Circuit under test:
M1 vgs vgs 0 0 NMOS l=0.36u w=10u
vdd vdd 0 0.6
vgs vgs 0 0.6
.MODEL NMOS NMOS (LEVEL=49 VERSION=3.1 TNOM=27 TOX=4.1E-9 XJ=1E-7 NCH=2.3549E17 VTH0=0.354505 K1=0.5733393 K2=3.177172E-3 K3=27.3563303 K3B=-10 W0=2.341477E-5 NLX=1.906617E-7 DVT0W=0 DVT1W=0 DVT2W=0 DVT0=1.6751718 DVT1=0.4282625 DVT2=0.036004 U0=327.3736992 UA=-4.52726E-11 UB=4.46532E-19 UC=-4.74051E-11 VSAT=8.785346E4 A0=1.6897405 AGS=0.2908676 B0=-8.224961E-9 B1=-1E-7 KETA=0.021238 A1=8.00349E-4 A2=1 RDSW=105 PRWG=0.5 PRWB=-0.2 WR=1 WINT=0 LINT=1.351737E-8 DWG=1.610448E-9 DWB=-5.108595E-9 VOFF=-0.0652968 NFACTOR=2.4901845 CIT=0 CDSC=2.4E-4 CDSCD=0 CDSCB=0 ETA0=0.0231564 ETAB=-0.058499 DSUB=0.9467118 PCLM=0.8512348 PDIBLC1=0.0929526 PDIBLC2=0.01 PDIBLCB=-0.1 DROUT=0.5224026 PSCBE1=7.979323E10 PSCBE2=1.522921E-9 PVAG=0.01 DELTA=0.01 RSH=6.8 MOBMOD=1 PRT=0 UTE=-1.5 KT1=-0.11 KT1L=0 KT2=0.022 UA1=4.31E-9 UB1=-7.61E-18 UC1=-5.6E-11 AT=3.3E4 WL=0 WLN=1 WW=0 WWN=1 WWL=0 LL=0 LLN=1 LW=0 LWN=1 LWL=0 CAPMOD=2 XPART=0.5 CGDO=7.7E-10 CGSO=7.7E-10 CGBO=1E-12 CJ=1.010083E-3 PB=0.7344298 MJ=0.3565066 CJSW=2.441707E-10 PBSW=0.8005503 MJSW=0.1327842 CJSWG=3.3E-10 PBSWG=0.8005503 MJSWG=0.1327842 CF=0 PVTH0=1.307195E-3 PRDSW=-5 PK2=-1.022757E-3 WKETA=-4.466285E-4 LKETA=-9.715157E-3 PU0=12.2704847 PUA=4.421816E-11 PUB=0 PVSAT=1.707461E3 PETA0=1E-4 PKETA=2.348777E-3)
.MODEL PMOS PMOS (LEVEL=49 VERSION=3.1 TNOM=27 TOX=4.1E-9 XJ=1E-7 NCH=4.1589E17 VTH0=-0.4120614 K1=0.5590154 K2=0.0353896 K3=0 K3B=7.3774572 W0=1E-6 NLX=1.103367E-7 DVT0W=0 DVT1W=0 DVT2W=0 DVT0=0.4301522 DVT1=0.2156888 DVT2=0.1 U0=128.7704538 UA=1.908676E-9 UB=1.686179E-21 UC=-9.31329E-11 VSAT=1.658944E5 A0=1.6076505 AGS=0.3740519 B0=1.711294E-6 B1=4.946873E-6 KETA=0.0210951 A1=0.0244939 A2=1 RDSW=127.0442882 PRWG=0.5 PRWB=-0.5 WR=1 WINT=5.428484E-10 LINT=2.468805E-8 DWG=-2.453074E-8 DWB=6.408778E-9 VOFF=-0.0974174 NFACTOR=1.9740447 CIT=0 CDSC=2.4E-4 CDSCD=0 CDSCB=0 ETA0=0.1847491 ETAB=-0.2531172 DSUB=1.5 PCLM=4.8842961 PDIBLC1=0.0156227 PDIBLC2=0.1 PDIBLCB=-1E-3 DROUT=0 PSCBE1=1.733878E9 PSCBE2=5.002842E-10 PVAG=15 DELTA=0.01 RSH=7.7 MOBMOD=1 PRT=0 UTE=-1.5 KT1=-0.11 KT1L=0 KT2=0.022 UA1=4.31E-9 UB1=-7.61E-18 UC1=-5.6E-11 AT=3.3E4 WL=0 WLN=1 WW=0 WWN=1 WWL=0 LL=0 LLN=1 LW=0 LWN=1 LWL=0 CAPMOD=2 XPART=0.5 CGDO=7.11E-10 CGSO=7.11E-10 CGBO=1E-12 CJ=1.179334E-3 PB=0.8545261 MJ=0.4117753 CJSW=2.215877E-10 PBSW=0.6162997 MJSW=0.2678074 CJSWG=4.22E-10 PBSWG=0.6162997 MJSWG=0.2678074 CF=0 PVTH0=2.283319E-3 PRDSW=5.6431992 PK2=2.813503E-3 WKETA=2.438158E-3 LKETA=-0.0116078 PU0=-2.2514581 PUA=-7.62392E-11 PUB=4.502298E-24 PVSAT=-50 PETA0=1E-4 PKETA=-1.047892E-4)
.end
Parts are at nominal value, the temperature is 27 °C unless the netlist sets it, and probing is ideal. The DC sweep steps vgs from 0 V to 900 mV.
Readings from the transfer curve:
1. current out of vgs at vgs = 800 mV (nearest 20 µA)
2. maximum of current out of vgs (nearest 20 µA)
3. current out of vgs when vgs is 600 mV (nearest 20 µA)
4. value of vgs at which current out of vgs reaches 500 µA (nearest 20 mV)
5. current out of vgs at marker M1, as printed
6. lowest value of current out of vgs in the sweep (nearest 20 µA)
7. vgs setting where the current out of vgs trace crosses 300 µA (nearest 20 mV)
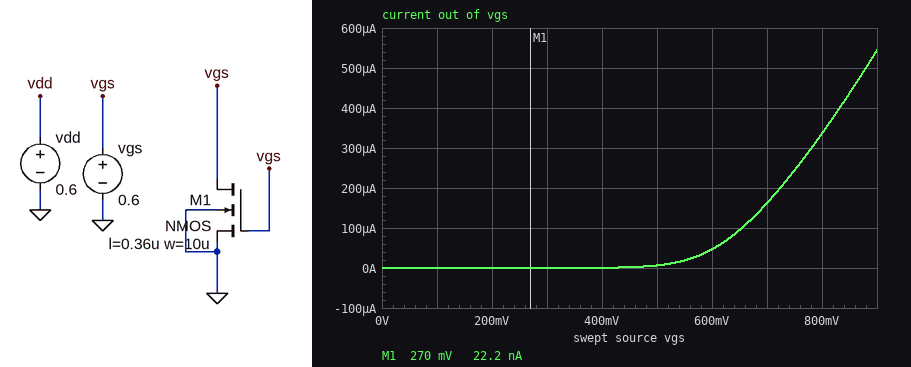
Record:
340 µA
540 µA
40 µA
880 mV
22.2 nA
0 A
780 mV
